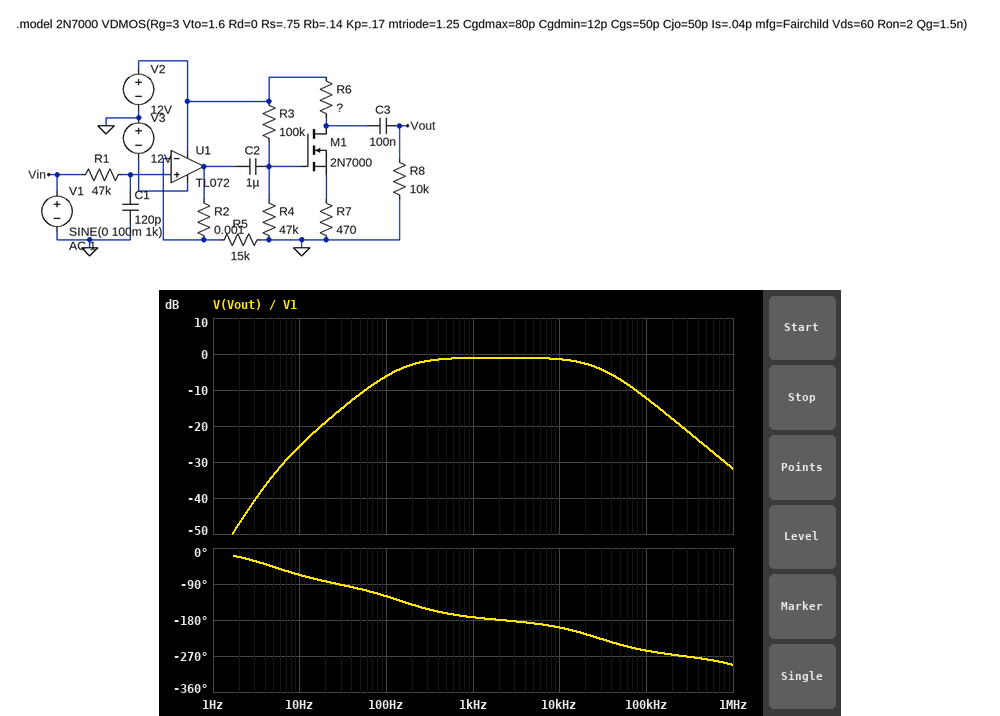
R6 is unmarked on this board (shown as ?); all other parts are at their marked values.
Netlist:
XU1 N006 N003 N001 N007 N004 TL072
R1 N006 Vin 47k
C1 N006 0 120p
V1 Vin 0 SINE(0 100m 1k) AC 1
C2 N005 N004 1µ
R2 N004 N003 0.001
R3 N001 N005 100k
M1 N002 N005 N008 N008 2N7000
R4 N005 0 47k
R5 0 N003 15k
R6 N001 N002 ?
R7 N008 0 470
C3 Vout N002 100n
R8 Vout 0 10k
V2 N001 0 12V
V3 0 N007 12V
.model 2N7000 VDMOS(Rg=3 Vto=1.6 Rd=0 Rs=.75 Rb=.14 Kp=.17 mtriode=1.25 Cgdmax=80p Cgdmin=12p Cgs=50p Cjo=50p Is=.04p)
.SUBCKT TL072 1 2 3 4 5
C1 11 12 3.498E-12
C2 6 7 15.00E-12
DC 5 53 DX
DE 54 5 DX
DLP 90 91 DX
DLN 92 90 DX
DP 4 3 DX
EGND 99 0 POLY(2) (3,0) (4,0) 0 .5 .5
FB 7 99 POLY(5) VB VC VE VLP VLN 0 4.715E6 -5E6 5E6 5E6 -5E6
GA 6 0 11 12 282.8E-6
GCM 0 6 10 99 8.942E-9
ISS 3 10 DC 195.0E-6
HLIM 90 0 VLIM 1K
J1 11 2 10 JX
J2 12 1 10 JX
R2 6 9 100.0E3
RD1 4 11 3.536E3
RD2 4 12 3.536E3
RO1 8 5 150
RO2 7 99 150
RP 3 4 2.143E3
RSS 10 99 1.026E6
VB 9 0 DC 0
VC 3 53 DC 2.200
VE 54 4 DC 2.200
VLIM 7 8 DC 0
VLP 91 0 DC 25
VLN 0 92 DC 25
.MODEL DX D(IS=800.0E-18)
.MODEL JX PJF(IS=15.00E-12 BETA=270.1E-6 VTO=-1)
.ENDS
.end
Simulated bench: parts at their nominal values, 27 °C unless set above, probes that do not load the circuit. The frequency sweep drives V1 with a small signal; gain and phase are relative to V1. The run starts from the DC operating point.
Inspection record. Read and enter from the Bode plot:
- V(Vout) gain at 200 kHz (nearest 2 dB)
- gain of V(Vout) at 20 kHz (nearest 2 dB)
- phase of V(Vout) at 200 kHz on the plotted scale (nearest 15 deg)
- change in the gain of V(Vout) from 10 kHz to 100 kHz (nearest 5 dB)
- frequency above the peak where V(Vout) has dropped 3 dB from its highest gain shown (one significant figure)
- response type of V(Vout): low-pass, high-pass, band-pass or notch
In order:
-18 dB
-2 dB
-270 deg
-10 dB
30 kHz
band-pass
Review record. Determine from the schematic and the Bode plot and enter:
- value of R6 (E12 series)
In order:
470 Ω
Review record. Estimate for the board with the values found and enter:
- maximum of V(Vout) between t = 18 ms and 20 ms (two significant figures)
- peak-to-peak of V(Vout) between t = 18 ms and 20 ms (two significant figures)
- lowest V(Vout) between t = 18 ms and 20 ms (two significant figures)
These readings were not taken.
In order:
89 mV
180 mV
-89 mV
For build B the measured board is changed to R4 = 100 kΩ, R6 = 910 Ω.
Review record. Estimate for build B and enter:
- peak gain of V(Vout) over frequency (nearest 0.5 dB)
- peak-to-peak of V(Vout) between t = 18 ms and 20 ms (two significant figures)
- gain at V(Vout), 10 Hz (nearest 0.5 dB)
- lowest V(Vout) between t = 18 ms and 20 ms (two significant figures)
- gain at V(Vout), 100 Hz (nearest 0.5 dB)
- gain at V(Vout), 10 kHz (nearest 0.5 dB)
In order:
-8.0 dB
120 mV
-32.0 dB
-42 mV
-13.0 dB
-8.5 dB
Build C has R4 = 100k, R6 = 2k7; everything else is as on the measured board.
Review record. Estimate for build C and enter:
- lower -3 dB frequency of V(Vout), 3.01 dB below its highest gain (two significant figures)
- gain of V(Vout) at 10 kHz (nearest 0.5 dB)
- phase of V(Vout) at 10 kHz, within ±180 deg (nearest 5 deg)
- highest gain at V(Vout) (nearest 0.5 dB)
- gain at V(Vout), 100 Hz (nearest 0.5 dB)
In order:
26 kHz
-49.0 dB
105 deg
-41.0 dB
-58.5 dB
